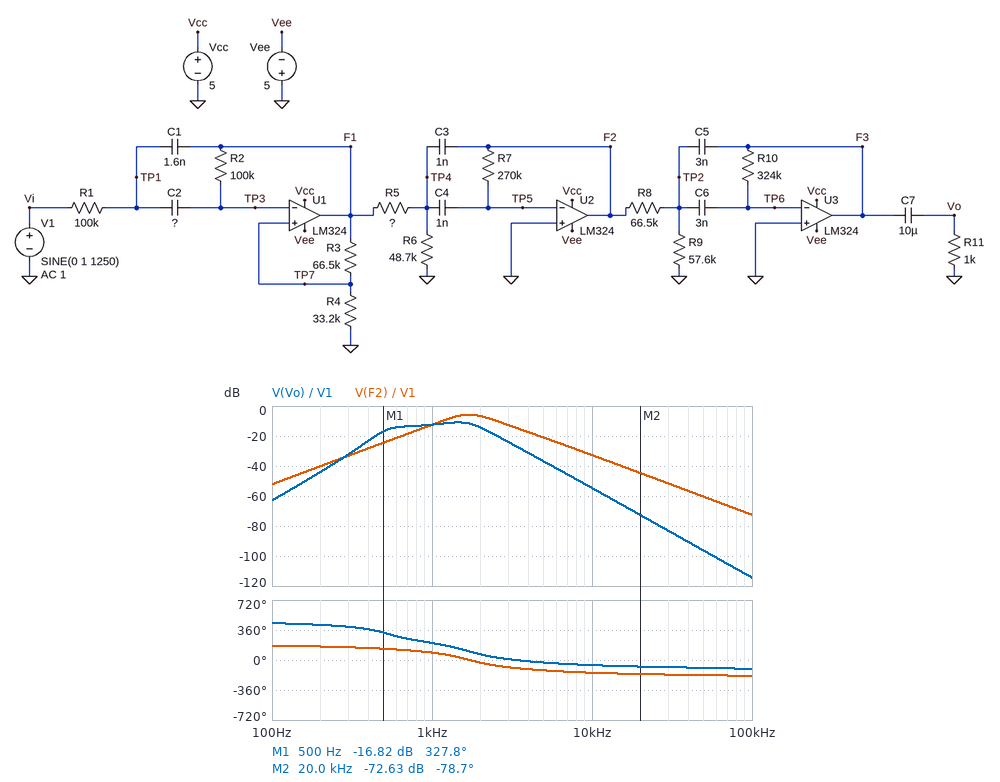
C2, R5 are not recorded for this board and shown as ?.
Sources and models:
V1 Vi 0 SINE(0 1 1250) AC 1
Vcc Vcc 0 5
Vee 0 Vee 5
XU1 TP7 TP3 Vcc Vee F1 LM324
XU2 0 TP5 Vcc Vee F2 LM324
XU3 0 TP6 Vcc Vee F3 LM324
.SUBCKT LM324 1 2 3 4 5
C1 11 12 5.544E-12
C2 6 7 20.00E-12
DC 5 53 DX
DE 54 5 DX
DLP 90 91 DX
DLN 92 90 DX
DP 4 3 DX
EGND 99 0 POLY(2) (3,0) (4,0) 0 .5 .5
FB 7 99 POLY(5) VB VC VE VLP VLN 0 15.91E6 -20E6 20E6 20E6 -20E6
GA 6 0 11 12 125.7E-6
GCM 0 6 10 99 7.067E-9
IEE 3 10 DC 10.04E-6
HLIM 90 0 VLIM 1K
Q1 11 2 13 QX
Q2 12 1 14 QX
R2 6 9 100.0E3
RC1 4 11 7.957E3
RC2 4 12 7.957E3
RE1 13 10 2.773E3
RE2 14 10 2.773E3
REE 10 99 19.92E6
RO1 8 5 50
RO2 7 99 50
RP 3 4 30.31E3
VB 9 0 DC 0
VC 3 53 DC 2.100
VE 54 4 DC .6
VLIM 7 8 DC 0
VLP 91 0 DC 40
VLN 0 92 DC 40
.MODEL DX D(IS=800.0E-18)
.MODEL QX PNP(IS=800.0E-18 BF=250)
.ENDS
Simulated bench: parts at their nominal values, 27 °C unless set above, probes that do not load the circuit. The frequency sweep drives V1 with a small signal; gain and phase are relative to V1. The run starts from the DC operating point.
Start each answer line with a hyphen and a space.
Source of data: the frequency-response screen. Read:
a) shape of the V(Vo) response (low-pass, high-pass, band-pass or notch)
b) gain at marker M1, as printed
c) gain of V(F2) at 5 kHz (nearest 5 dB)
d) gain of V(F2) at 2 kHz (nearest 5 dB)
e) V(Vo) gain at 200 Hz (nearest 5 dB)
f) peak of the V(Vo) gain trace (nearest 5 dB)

- band-pass
- -16.82 dB
- -20 dB
- -5 dB
- -45 dB
- -10 dB
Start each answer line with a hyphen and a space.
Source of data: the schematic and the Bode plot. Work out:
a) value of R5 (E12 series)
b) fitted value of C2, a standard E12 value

- 100 kΩ
- 470 pF
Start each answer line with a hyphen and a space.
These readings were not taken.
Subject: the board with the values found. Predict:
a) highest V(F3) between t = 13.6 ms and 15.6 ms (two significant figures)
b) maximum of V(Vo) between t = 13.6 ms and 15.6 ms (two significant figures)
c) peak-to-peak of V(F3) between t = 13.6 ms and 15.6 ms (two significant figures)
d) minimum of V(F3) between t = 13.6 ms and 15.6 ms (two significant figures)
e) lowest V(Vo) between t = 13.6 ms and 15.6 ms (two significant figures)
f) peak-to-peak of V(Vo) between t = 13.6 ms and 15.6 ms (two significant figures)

- 260 mV
- 270 mV
- 540 mV
- -280 mV
- -270 mV
- 540 mV
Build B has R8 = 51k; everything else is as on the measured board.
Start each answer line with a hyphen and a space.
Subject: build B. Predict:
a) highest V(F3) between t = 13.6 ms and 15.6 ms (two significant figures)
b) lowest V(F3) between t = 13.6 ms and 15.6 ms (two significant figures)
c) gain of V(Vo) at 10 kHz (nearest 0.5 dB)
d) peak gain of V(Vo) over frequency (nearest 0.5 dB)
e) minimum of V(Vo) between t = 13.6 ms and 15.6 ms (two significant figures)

- 360 mV
- -370 mV
- -52.5 dB
- -8.5 dB
- -360 mV
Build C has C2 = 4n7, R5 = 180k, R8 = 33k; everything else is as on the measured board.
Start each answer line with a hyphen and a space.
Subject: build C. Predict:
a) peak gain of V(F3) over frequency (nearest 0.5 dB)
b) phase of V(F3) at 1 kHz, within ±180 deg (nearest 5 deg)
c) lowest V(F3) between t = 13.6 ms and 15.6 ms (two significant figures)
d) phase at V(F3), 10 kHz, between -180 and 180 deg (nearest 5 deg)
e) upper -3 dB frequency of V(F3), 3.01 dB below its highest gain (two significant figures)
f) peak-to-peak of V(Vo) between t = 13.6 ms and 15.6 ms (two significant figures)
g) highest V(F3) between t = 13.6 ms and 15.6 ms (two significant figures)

- 7.5 dB
- 130 deg
- -1.2 V
- -80 deg
- 960 Hz
- 2.4 V
- 1.2 V
